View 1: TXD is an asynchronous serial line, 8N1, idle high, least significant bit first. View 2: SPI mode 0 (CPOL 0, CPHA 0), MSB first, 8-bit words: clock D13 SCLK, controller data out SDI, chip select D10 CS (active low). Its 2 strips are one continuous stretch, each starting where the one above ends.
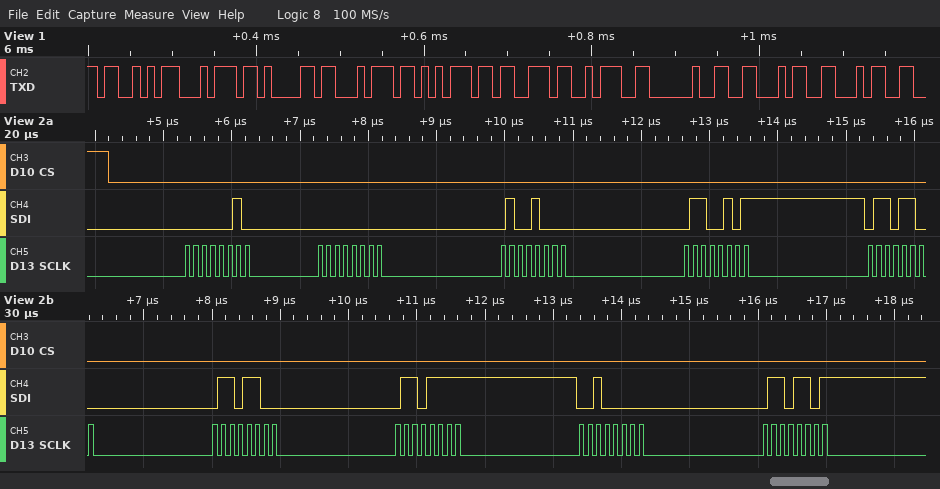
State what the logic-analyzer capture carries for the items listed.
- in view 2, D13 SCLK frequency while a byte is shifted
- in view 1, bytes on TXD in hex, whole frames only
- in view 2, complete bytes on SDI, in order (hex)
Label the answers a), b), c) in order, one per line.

a) 8 MHz
b) 53 74 61 74 75 73 3A 20 46 46
c) 02 00 48 65 6C 6C 6F 20 6D
